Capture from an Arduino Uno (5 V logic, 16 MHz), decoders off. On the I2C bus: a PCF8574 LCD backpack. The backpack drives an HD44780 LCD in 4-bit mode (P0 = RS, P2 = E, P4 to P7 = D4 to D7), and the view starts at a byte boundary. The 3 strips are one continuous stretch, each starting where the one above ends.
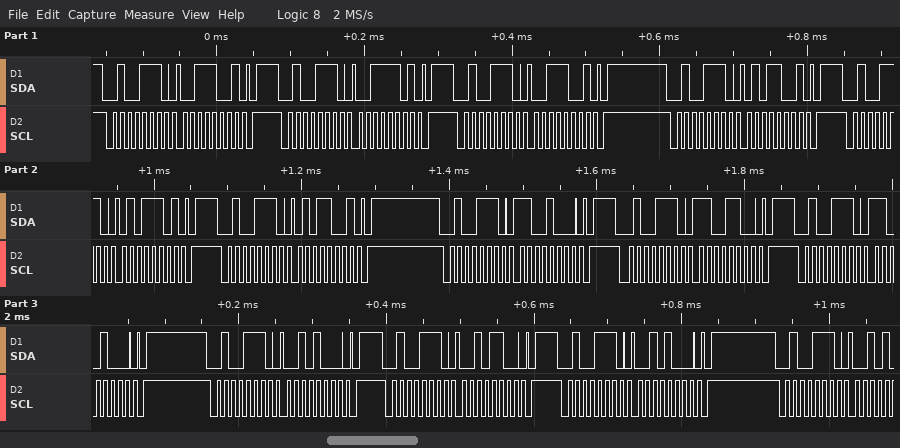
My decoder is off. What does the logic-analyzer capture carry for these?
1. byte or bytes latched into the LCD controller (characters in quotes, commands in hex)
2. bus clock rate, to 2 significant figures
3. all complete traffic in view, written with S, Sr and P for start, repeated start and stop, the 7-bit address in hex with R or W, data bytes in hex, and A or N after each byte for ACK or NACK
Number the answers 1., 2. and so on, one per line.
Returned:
1. '5' 0xC2
2. 100 kHz
3. S 27W A 39 A P S 27W A 3D A P S 27W A 39 A P S 27W A 59 A P S 27W A 5D A P S 27W A 59 A P S 27W A C8 A P S 27W A CC A P S 27W A C8 A P S 27W A 28 A P S 27W A 2C A P S 27W A 28 A P S 27W A
